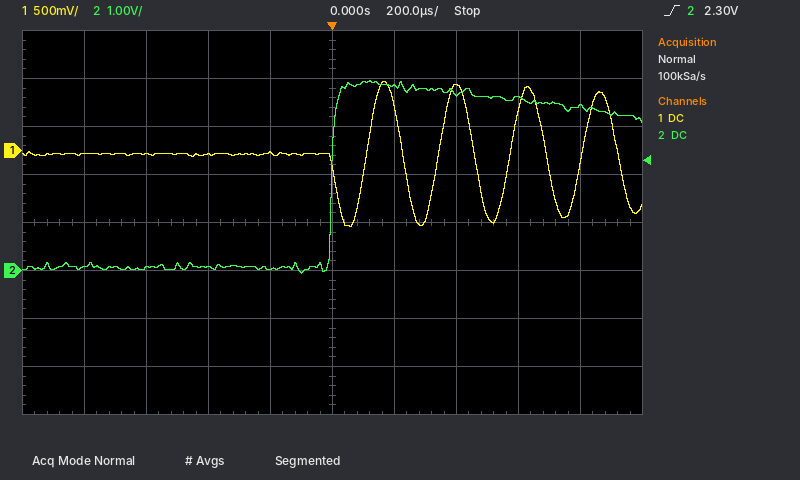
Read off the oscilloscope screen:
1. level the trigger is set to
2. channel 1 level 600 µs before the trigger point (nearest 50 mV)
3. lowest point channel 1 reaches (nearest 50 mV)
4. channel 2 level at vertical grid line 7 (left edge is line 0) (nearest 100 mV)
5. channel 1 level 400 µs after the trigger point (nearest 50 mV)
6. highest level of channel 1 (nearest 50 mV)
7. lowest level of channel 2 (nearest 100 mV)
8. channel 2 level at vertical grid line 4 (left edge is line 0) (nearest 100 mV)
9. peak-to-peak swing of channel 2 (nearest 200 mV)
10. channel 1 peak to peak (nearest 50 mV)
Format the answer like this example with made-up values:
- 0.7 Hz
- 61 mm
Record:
- 2.30 V
- -50 mV
- -800 mV
- 3.7 V
- 700 mV
- 700 mV
- -100 mV
- 0.0 V
- 4.0 V
- 1.50 V
